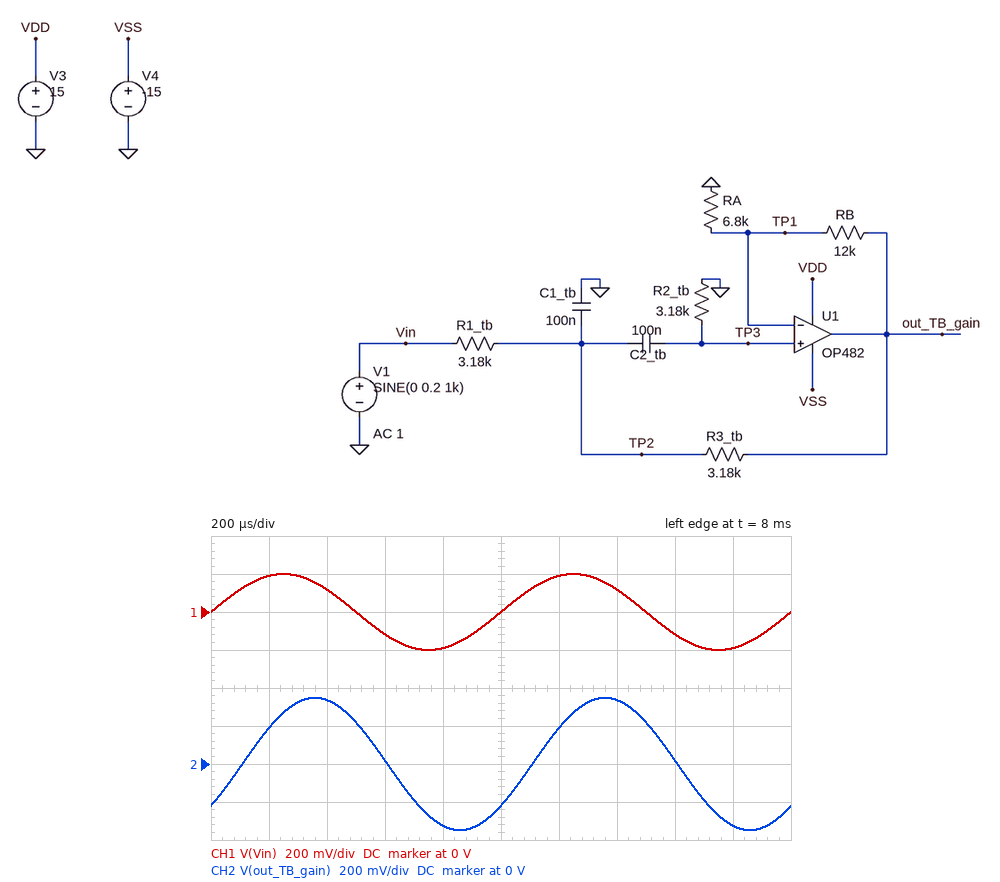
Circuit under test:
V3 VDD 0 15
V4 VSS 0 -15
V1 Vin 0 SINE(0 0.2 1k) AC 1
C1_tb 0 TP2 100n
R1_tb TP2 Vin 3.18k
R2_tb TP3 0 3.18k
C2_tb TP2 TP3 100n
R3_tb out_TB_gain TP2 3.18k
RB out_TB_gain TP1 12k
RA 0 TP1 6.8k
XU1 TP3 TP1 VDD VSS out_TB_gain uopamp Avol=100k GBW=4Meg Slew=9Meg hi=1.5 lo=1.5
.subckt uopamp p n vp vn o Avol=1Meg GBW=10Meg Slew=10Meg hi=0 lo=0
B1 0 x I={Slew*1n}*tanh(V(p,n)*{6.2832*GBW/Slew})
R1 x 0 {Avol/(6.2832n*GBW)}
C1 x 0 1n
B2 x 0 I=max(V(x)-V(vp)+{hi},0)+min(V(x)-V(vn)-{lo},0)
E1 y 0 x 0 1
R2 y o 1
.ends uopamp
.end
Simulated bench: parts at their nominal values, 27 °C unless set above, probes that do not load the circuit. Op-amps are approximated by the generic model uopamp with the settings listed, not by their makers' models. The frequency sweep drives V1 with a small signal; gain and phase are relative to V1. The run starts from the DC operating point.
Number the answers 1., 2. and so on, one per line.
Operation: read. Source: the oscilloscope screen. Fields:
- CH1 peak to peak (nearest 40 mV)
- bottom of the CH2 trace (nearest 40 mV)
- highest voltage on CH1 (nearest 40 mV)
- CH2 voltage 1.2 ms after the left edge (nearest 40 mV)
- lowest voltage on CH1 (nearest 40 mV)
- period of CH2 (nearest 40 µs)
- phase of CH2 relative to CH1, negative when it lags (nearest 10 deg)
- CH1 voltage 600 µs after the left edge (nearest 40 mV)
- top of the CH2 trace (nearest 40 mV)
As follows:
1. 400 mV
2. -360 mV
3. 200 mV
4. 200 mV
5. -200 mV
6. 1.00 ms
7. -40 deg
8. -120 mV
9. 360 mV
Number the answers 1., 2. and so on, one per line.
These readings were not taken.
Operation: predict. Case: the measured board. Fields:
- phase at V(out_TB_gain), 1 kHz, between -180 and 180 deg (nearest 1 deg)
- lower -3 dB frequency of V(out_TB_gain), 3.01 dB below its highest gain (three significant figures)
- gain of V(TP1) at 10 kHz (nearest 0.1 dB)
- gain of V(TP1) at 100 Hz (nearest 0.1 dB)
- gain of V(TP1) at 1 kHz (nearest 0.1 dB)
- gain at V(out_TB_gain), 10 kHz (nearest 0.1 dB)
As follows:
1. -39 deg
2. 463 Hz
3. -26.0 dB
4. -19.9 dB
5. -4.0 dB
6. -17.2 dB
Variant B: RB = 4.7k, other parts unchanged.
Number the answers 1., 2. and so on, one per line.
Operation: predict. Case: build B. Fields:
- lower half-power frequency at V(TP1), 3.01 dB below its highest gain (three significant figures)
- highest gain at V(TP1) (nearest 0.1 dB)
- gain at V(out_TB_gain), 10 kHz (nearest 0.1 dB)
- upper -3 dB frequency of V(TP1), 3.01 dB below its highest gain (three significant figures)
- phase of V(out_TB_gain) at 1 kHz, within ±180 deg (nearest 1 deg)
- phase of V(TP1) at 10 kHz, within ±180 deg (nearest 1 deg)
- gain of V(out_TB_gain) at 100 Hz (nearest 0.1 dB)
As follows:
1. 336 Hz
2. -7.3 dB
3. -21.5 dB
4. 1.49 kHz
5. -23 deg
6. -84 deg
7. -15.5 dB
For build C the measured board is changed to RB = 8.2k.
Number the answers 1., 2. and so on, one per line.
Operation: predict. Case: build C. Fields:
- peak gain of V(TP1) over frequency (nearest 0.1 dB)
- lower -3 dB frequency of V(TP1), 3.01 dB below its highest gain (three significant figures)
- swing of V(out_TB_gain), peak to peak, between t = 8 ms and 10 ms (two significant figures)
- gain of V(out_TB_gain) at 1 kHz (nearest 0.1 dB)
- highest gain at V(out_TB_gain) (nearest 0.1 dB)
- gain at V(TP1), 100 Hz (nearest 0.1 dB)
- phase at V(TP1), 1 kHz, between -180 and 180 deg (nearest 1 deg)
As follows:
1. -5.1 dB
2. 389 Hz
3. 430 mV
4. 0.6 dB
5. 1.8 dB
6. -20.0 dB
7. -29 deg
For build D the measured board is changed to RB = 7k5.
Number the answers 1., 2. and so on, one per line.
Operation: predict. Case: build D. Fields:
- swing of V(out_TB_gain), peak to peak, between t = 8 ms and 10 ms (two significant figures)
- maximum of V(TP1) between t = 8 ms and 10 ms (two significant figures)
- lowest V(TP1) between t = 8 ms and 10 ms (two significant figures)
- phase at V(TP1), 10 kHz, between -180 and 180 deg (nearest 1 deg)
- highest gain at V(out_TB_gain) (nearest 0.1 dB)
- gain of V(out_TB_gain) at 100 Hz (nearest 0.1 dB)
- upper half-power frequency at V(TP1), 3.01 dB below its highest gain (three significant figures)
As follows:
1. 390 mV
2. 93 mV
3. -93 mV
4. -85 deg
5. 0.9 dB
6. -13.5 dB
7. 1.33 kHz
